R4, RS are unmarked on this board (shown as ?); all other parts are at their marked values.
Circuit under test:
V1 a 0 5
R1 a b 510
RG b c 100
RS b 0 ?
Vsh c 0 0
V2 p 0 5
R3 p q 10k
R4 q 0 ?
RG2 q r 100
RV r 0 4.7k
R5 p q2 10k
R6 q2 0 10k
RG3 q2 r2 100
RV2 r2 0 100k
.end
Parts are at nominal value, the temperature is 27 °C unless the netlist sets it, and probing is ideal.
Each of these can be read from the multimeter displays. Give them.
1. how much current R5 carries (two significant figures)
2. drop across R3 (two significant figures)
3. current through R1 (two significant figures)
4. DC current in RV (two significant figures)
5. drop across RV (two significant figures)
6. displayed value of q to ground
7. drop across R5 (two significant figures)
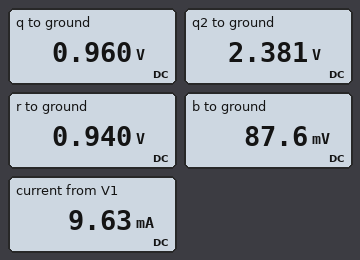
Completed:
260 µA
4.0 V
9.6 mA
200 µA
940 mV
0.960 V
2.6 V
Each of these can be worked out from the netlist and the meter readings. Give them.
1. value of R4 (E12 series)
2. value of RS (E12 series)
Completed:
4.7 kΩ
10 Ω
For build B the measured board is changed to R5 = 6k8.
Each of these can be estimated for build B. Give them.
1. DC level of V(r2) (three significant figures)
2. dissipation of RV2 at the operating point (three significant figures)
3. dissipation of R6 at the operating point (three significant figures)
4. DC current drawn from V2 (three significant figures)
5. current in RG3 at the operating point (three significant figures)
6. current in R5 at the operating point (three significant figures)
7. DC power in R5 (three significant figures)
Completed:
2.86 V
81.7 µW
818 µW
719 µA
28.6 µA
315 µA
673 µW
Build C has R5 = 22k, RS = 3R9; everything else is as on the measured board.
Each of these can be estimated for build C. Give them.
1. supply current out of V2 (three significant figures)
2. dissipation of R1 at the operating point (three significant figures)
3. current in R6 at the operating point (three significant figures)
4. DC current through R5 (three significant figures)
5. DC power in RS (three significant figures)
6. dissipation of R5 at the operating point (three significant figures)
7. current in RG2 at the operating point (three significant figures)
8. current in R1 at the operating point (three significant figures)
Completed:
565 µA
48.3 mW
146 µA
161 µA
342 µW
569 µW
200 µA
9.73 mA
